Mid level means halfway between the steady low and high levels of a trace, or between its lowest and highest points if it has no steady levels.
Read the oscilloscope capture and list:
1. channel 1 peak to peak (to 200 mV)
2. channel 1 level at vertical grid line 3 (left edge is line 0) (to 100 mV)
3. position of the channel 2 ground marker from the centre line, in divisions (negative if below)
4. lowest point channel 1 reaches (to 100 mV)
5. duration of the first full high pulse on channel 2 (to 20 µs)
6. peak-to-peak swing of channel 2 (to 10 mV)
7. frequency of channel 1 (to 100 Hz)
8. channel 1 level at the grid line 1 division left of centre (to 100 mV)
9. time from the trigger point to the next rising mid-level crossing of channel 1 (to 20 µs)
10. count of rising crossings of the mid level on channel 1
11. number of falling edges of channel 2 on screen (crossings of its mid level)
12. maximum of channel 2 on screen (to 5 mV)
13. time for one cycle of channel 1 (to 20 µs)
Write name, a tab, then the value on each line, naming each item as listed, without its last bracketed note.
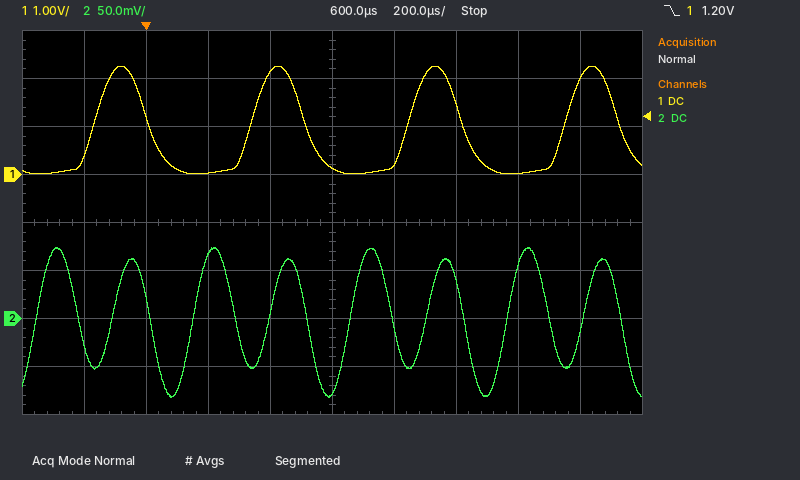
channel 1 peak to peak	2.2 V
channel 1 level at vertical grid line 3 (left edge is line 0)	0.0 V
position of the channel 2 ground marker from the centre line, in divisions	-2.0 div
lowest point channel 1 reaches	0.0 V
duration of the first full high pulse on channel 2	140 µs
peak-to-peak swing of channel 2	160 mV
frequency of channel 1	2.0 kHz
channel 1 level at the grid line 1 division left of centre	2.1 V
time from the trigger point to the next rising mid-level crossing of channel 1	340 µs
count of rising crossings of the mid level on channel 1	4
number of falling edges of channel 2 on screen	8
maximum of channel 2 on screen	75 mV
time for one cycle of channel 1	500 µs
